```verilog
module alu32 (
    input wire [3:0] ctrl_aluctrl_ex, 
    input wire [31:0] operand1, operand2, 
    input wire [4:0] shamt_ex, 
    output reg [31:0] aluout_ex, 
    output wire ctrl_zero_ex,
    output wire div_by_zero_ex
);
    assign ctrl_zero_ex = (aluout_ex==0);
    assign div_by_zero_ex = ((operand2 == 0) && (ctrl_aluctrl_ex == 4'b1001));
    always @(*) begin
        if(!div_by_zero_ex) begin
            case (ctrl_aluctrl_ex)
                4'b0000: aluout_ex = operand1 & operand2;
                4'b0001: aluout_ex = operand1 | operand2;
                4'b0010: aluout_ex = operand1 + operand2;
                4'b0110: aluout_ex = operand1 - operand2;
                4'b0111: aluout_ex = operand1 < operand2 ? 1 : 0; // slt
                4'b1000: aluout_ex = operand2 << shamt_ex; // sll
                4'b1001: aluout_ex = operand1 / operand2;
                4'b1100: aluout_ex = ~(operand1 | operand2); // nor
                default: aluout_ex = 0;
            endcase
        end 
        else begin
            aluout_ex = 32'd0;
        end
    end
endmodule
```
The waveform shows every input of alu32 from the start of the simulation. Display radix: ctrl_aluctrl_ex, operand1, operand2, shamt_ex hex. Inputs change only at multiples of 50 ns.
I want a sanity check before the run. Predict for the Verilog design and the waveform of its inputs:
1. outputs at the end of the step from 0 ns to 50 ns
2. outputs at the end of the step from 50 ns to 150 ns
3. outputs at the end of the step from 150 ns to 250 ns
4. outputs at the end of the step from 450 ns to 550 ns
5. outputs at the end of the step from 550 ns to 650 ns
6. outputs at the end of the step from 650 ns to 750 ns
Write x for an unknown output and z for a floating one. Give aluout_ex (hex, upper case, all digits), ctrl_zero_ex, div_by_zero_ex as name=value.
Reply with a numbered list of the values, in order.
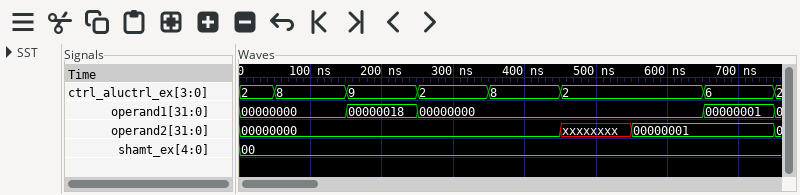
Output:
1. aluout_ex=00000000, ctrl_zero_ex=1, div_by_zero_ex=0
2. aluout_ex=00000000, ctrl_zero_ex=1, div_by_zero_ex=0
3. aluout_ex=00000000, ctrl_zero_ex=1, div_by_zero_ex=1
4. aluout_ex=x, ctrl_zero_ex=x, div_by_zero_ex=0
5. aluout_ex=00000001, ctrl_zero_ex=0, div_by_zero_ex=0
6. aluout_ex=00000000, ctrl_zero_ex=1, div_by_zero_ex=0
